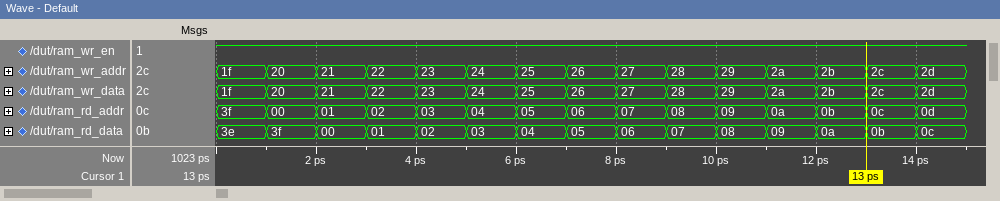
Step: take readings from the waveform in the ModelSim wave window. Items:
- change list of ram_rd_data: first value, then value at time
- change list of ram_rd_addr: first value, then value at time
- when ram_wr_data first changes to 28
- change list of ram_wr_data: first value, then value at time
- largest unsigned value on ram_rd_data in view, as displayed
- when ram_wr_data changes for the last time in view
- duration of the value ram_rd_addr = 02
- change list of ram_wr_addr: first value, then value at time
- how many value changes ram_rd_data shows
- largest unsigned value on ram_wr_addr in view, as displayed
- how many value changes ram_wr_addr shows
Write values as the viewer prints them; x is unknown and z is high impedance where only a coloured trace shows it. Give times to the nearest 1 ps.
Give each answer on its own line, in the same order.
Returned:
3e, 3f at 1 ps, 00 at 2 ps, 01 at 3 ps, 02 at 4 ps, 03 at 5 ps, 04 at 6 ps, 05 at 7 ps, 06 at 8 ps, 07 at 9 ps, 08 at 10 ps, 09 at 11 ps, 0a at 12 ps, 0b at 13 ps, 0c at 14 ps
3f, 00 at 1 ps, 01 at 2 ps, 02 at 3 ps, 03 at 4 ps, 04 at 5 ps, 05 at 6 ps, 06 at 7 ps, 07 at 8 ps, 08 at 9 ps, 09 at 10 ps, 0a at 11 ps, 0b at 12 ps, 0c at 13 ps, 0d at 14 ps
9 ps
1f, 20 at 1 ps, 21 at 2 ps, 22 at 3 ps, 23 at 4 ps, 24 at 5 ps, 25 at 6 ps, 26 at 7 ps, 27 at 8 ps, 28 at 9 ps, 29 at 10 ps, 2a at 11 ps, 2b at 12 ps, 2c at 13 ps, 2d at 14 ps
3f
14 ps
1 ps
1f, 20 at 1 ps, 21 at 2 ps, 22 at 3 ps, 23 at 4 ps, 24 at 5 ps, 25 at 6 ps, 26 at 7 ps, 27 at 8 ps, 28 at 9 ps, 29 at 10 ps, 2a at 11 ps, 2b at 12 ps, 2c at 13 ps, 2d at 14 ps
14
2d
14
